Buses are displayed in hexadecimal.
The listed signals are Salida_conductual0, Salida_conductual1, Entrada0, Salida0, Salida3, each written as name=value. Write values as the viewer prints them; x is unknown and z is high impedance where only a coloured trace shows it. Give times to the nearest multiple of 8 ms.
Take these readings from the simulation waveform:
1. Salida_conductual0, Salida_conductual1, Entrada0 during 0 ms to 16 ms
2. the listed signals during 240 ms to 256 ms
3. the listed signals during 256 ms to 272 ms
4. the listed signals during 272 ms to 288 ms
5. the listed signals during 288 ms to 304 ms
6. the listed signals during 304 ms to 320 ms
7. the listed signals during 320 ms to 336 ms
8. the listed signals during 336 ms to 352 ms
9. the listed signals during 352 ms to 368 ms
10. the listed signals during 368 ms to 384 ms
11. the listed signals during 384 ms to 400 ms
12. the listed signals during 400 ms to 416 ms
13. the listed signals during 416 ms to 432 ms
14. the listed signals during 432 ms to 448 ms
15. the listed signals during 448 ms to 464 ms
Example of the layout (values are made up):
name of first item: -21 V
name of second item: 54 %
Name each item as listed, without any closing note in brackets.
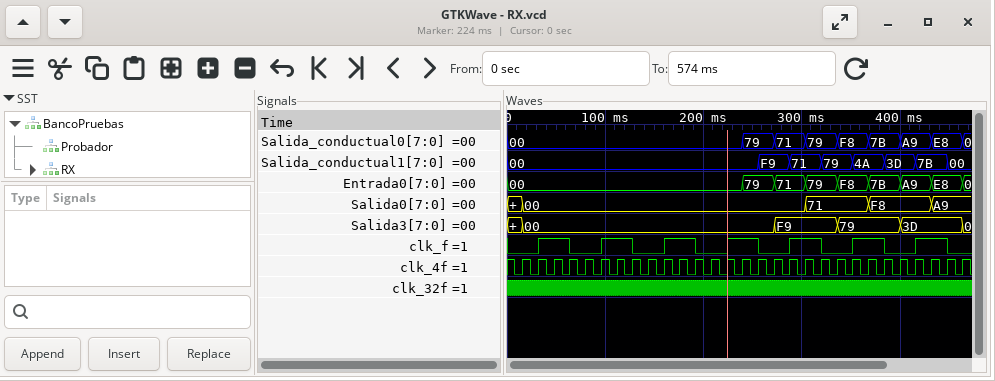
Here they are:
Salida_conductual0, Salida_conductual1, Entrada0 during 0 ms to 16 ms: Salida_conductual0=00, Salida_conductual1=00, Entrada0=00
the listed signals during 240 ms to 256 ms: Salida_conductual0=79, Salida_conductual1=00, Entrada0=79, Salida0=00, Salida3=00
the listed signals during 256 ms to 272 ms: Salida_conductual0=79, Salida_conductual1=F9, Entrada0=79, Salida0=00, Salida3=00
the listed signals during 272 ms to 288 ms: Salida_conductual0=71, Salida_conductual1=F9, Entrada0=71, Salida0=00, Salida3=F9
the listed signals during 288 ms to 304 ms: Salida_conductual0=71, Salida_conductual1=71, Entrada0=71, Salida0=00, Salida3=F9
the listed signals during 304 ms to 320 ms: Salida_conductual0=79, Salida_conductual1=71, Entrada0=79, Salida0=71, Salida3=F9
the listed signals during 320 ms to 336 ms: Salida_conductual0=79, Salida_conductual1=79, Entrada0=79, Salida0=71, Salida3=F9
the listed signals during 336 ms to 352 ms: Salida_conductual0=F8, Salida_conductual1=79, Entrada0=F8, Salida0=71, Salida3=79
the listed signals during 352 ms to 368 ms: Salida_conductual0=F8, Salida_conductual1=4A, Entrada0=F8, Salida0=71, Salida3=79
the listed signals during 368 ms to 384 ms: Salida_conductual0=7B, Salida_conductual1=4A, Entrada0=7B, Salida0=F8, Salida3=79
the listed signals during 384 ms to 400 ms: Salida_conductual0=7B, Salida_conductual1=3D, Entrada0=7B, Salida0=F8, Salida3=79
the listed signals during 400 ms to 416 ms: Salida_conductual0=A9, Salida_conductual1=3D, Entrada0=A9, Salida0=F8, Salida3=3D
the listed signals during 416 ms to 432 ms: Salida_conductual0=A9, Salida_conductual1=7B, Entrada0=A9, Salida0=F8, Salida3=3D
the listed signals during 432 ms to 448 ms: Salida_conductual0=E8, Salida_conductual1=7B, Entrada0=E8, Salida0=A9, Salida3=3D
the listed signals during 448 ms to 464 ms: Salida_conductual0=E8, Salida_conductual1=00, Entrada0=E8, Salida0=A9, Salida3=3D
